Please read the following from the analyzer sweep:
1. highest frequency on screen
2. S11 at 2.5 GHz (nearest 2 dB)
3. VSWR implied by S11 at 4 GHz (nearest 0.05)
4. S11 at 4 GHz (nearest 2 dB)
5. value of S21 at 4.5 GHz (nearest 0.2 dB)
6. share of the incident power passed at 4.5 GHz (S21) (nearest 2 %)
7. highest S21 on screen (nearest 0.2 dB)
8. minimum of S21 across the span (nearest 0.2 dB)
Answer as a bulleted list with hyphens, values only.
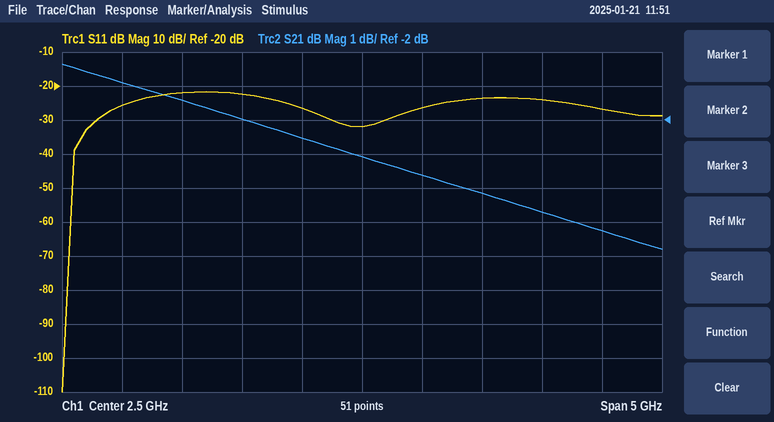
- 5 GHz
- -32 dB
- 1.15
- -24 dB
- -5.2 dB
- 30 %
- -0.4 dB
- -5.8 dB
